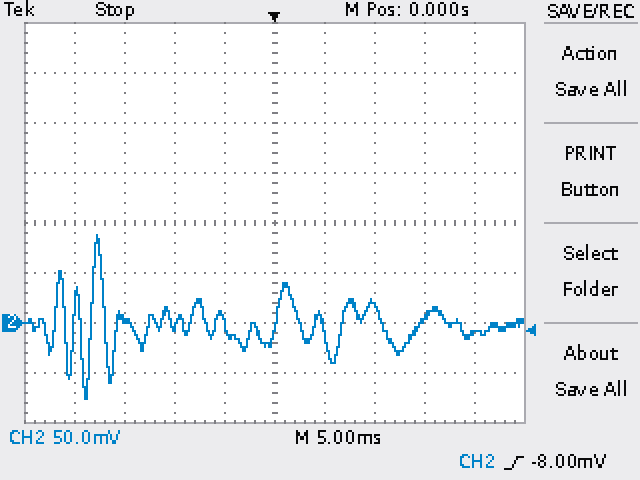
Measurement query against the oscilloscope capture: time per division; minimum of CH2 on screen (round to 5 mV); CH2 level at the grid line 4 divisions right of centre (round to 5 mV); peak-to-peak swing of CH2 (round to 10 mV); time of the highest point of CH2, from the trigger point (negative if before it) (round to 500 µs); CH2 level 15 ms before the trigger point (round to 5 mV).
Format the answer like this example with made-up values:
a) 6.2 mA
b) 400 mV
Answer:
a) 5 ms
b) -75 mV
c) -10 mV
d) 160 mV
e) -17.5 ms
f) 5 mV
